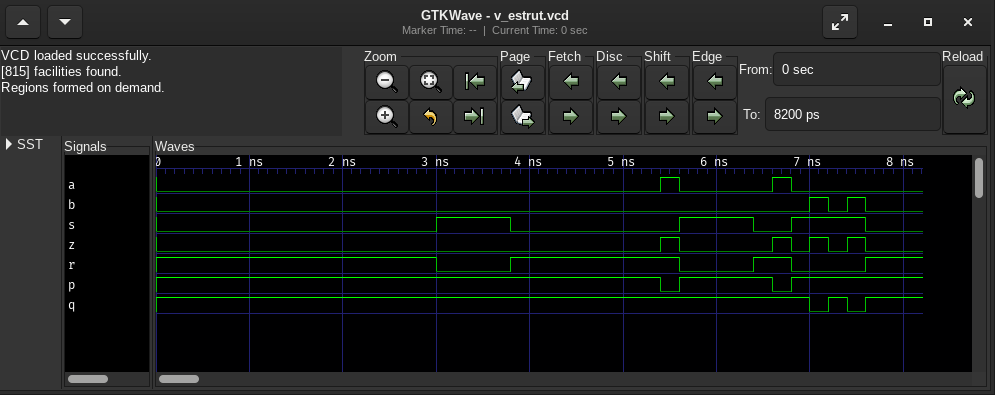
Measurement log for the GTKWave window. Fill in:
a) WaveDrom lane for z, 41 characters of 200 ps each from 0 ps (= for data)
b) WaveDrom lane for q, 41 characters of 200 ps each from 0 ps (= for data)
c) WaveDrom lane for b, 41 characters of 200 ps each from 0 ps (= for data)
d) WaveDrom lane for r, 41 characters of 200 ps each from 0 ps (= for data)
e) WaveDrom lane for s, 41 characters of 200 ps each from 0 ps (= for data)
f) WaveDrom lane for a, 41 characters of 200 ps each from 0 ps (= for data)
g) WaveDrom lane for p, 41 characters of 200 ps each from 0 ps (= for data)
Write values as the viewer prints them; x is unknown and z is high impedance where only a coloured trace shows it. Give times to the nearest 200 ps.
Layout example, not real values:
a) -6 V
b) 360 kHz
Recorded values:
a) {name: 'z', wave: '0..........................10....101010..'}
b) {name: 'q', wave: '1..................................0101..'}
c) {name: 'b', wave: '0..................................1010..'}
d) {name: 'r', wave: '1..............0...1........0...1.0...1..'}
e) {name: 's', wave: '0..............1...0........1...0.1...0..'}
f) {name: 'a', wave: '0..........................10....10......'}
g) {name: 'p', wave: '1..........................01....01......'}
